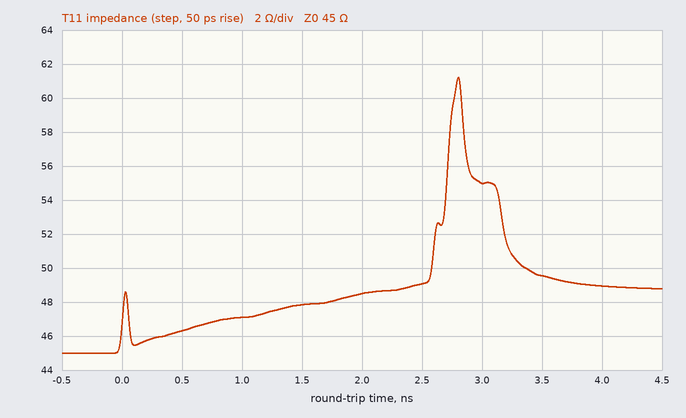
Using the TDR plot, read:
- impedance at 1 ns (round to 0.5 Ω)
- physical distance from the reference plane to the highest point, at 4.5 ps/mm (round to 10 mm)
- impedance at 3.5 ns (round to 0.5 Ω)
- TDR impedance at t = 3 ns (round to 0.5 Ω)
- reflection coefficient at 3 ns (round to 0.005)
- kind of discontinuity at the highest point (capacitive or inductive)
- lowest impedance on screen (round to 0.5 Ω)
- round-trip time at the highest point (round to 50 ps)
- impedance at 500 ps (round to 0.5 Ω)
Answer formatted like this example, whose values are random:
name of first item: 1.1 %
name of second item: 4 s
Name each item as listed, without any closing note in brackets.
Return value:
impedance at 1 ns: 47.0 Ω
physical distance from the reference plane to the highest point, at 4.5 ps/mm: 310 mm
impedance at 3.5 ns: 49.5 Ω
TDR impedance at t = 3 ns: 55.0 Ω
reflection coefficient at 3 ns: +0.100
kind of discontinuity at the highest point: inductive
lowest impedance on screen: 45.0 Ω
round-trip time at the highest point: 2.80 ns
impedance at 500 ps: 46.5 Ω
